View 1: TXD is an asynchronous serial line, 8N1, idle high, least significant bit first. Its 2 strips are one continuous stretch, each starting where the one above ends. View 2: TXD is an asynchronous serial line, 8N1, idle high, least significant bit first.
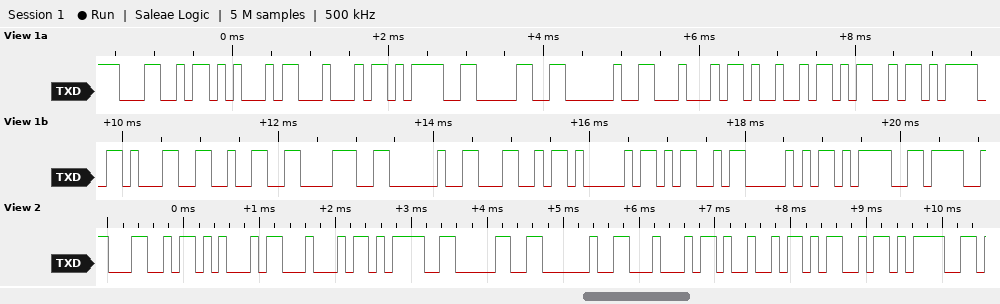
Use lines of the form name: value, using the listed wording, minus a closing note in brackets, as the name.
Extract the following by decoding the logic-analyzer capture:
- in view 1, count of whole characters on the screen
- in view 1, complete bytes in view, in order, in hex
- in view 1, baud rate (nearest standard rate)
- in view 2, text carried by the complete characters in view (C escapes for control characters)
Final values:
in view 1, count of whole characters on the screen: 19
in view 1, complete bytes in view, in order, in hex: 4C 45 44 3D 30 20 44 49 4D 3D 31 32 38 20 4C 41 4D 50 3D
in view 1, baud rate: 9600 baud
in view 2, text carried by the complete characters in view: "LED=0 DIM="
